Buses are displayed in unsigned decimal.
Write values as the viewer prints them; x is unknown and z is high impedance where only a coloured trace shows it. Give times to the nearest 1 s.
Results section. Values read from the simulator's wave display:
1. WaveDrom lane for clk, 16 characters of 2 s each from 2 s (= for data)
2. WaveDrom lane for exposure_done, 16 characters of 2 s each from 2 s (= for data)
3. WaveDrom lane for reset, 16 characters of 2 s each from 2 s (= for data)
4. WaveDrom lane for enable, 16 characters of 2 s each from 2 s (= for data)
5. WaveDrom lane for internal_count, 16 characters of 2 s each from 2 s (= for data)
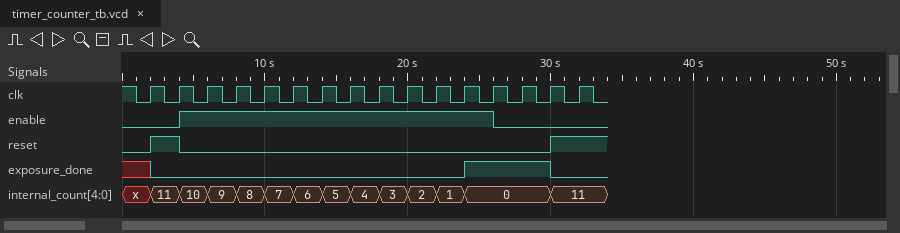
{name: 'clk', wave: 'p...............'}
{name: 'exposure_done', wave: '0..........1..0.'}
{name: 'reset', wave: '10............1.'}
{name: 'enable', wave: '01..........0...'}
{name: 'internal_count', wave: '============..=.', data: '11 10 9 8 7 6 5 4 3 2 1 0 11'}
